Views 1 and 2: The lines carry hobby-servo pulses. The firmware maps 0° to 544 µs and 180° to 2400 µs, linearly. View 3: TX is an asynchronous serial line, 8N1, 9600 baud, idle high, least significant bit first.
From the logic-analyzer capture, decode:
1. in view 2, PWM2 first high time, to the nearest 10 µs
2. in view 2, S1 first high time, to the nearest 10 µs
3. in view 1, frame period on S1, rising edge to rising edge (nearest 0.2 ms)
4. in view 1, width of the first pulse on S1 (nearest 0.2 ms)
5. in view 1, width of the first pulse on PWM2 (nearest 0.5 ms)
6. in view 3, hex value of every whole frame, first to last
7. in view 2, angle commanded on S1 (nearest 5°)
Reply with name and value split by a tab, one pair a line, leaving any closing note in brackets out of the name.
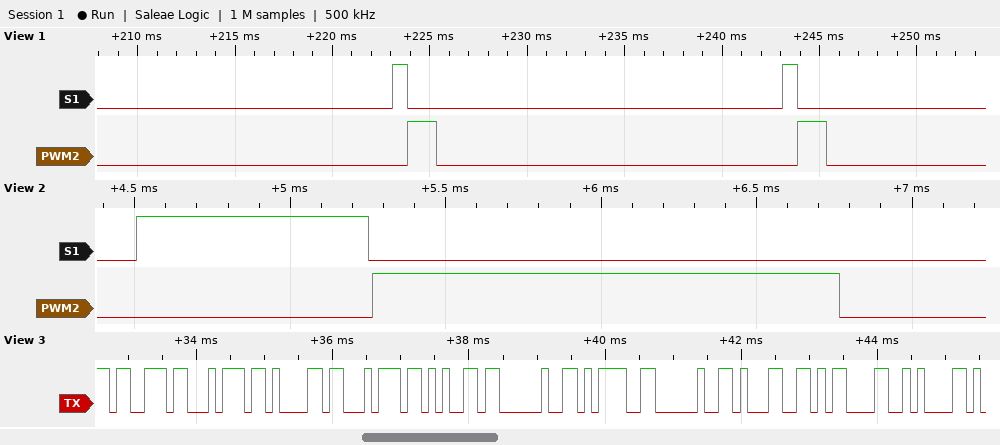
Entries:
in view 2, PWM2 first high time, to the nearest 10 µs	1500 µs
in view 2, S1 first high time, to the nearest 10 µs	750 µs
in view 1, frame period on S1, rising edge to rising edge	20.0 ms
in view 1, width of the first pulse on S1	0.8 ms
in view 1, width of the first pulse on PWM2	1.5 ms
in view 3, hex value of every whole frame, first to last	73 74 61 74 65 20 3D 20 31 0D 0A
in view 2, angle commanded on S1	20°
